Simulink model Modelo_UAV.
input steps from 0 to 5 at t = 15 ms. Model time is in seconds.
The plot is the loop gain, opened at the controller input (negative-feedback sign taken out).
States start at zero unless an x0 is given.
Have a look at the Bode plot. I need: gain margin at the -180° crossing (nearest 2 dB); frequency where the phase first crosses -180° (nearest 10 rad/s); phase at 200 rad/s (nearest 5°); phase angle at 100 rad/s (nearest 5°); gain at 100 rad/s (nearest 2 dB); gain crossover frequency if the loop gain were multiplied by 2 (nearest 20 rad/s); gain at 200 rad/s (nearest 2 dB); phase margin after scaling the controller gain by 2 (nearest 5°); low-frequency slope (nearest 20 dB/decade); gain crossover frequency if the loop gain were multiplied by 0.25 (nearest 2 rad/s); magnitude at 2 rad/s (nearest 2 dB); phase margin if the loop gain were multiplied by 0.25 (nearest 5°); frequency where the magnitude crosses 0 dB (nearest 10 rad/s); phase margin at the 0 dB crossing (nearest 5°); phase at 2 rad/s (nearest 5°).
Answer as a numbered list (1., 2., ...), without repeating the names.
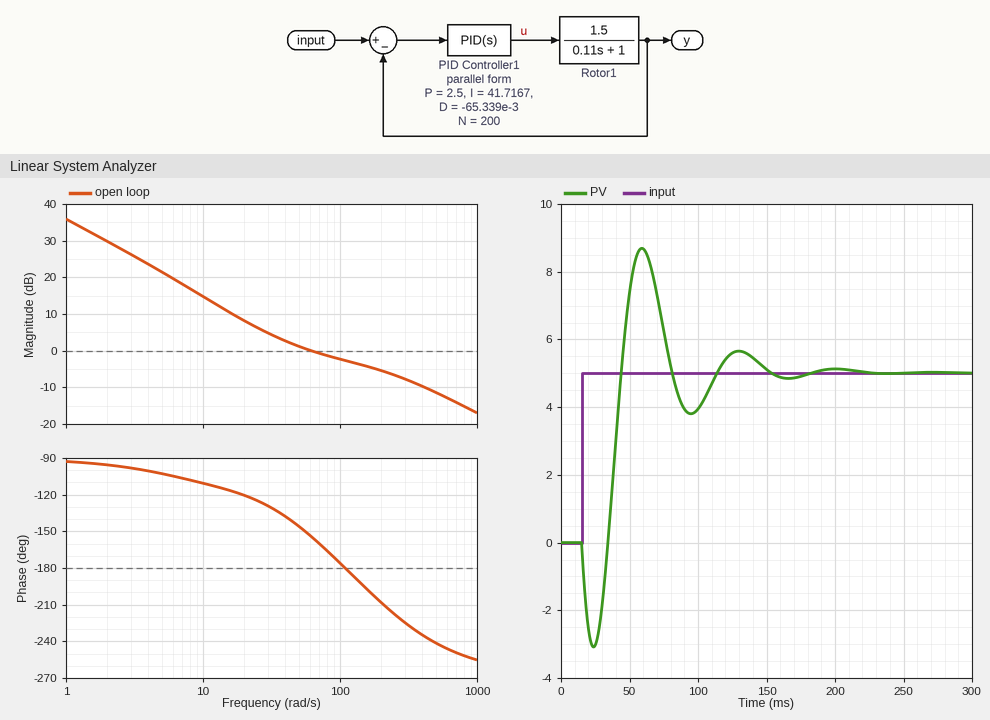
1. 2 dB
2. 110 rad/s
3. -210°
4. -175°
5. -2 dB
6. 220 rad/s
7. -6 dB
8. -35°
9. -20 dB/decade
10. 14 rad/s
11. 30 dB
12. 65°
13. 60 rad/s
14. 25°
15. -95°
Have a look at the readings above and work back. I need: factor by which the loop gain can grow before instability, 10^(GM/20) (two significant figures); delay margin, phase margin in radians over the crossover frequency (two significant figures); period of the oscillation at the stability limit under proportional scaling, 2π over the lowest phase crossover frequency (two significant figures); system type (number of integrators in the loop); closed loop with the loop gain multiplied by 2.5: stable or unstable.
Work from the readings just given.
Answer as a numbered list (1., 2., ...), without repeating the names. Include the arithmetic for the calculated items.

1. 10^(2 / 20) = 1.3
2. 25 × π / 180 / 60 = 0.0073 s
3. 2π / 110 = 0.057 s
4. 1
5. unstable
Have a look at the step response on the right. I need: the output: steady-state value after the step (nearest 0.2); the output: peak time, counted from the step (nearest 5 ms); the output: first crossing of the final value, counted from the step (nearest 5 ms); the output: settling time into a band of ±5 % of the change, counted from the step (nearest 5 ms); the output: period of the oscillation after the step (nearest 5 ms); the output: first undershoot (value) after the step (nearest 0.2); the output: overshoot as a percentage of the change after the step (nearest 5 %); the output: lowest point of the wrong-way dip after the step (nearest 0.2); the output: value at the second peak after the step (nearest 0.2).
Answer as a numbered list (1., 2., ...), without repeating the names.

1. 5.0
2. 45 ms
3. 30 ms
4. 130 ms
5. 70 ms
6. 3.8
7. 75 %
8. -3.0
9. 5.6
